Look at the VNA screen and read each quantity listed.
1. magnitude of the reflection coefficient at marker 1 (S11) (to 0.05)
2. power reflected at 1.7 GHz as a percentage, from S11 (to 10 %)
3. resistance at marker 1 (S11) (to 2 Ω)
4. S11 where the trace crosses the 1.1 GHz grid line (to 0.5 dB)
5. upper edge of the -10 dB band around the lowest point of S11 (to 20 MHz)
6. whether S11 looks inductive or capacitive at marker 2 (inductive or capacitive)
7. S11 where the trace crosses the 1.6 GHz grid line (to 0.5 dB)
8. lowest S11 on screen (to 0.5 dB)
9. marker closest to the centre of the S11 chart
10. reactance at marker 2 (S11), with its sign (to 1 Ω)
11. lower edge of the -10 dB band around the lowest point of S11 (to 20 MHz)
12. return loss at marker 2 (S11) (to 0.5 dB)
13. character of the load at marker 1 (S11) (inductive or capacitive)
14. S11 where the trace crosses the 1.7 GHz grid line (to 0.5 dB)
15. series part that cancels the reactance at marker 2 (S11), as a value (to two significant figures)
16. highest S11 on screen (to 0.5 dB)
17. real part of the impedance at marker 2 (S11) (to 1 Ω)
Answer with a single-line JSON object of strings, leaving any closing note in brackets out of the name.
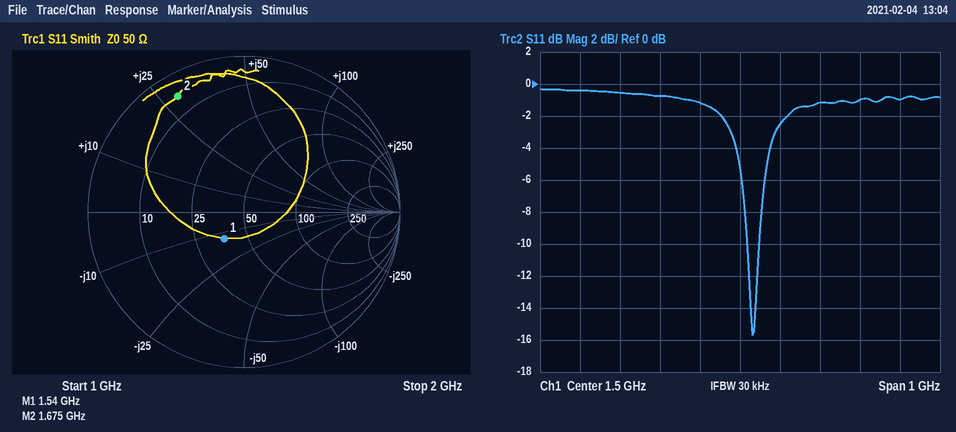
{"magnitude of the reflection coefficient at marker 1 (S11)": "0.20", "power reflected at 1.7 GHz as a percentage, from S11": "80 %", "resistance at marker 1 (S11)": "36 Ω", "S11 where the trace crosses the 1.1 GHz grid line": "-0.5 dB", "upper edge of the -10 dB band around the lowest point of S11": "1.54 GHz", "whether S11 looks inductive or capacitive at marker 2": "inductive", "S11 where the trace crosses the 1.6 GHz grid line": "-2.5 dB", "lowest S11 on screen": "-15.5 dB", "marker closest to the centre of the S11 chart": "marker 1", "reactance at marker 2 (S11), with its sign": "+29 Ω", "lower edge of the -10 dB band around the lowest point of S11": "1.52 GHz", "return loss at marker 2 (S11)": "1.5 dB", "character of the load at marker 1 (S11)": "capacitive", "S11 where the trace crosses the 1.7 GHz grid line": "-1.0 dB", "series part that cancels the reactance at marker 2 (S11), as a value": "3.3 pF", "highest S11 on screen": "-0.5 dB", "real part of the impedance at marker 2 (S11)": "5 Ω"}
